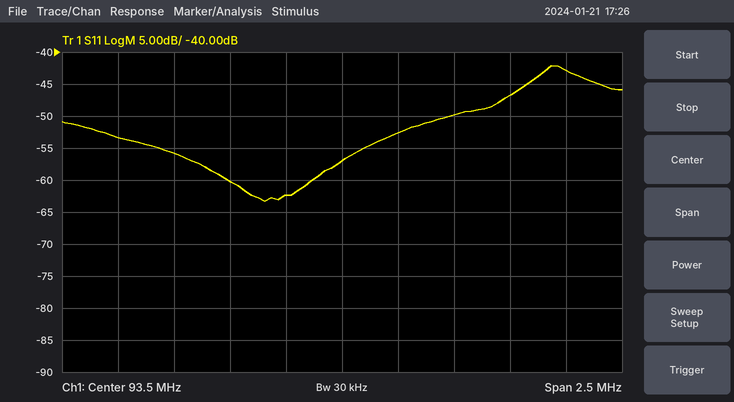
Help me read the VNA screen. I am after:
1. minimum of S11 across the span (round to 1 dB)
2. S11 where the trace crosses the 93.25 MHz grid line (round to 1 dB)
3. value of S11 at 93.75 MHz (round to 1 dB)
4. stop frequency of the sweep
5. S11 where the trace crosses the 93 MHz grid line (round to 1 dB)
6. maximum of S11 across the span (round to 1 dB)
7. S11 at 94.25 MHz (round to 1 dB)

-63 dB
-62 dB
-53 dB
94.75 MHz
-60 dB
-42 dB
-47 dB
